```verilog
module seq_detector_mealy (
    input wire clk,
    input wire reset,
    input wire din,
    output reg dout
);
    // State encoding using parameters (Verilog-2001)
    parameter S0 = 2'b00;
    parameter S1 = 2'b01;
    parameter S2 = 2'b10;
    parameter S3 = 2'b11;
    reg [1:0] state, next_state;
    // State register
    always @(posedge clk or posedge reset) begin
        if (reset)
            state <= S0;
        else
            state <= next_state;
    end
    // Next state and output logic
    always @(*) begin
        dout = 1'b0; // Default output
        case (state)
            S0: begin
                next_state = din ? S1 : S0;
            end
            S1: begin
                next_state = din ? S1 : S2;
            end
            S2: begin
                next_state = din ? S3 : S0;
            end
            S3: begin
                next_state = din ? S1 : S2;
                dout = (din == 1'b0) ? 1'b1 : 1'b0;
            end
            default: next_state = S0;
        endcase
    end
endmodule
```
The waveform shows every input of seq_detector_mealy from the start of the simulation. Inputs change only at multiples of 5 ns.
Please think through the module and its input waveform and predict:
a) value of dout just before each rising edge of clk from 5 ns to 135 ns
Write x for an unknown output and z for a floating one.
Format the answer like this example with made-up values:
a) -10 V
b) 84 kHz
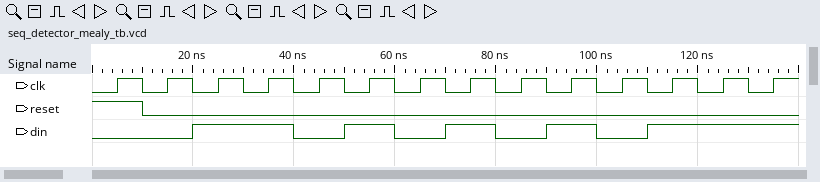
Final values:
a) 0 0 0 0 0 0 1 0 1 0 1 0 0 0
